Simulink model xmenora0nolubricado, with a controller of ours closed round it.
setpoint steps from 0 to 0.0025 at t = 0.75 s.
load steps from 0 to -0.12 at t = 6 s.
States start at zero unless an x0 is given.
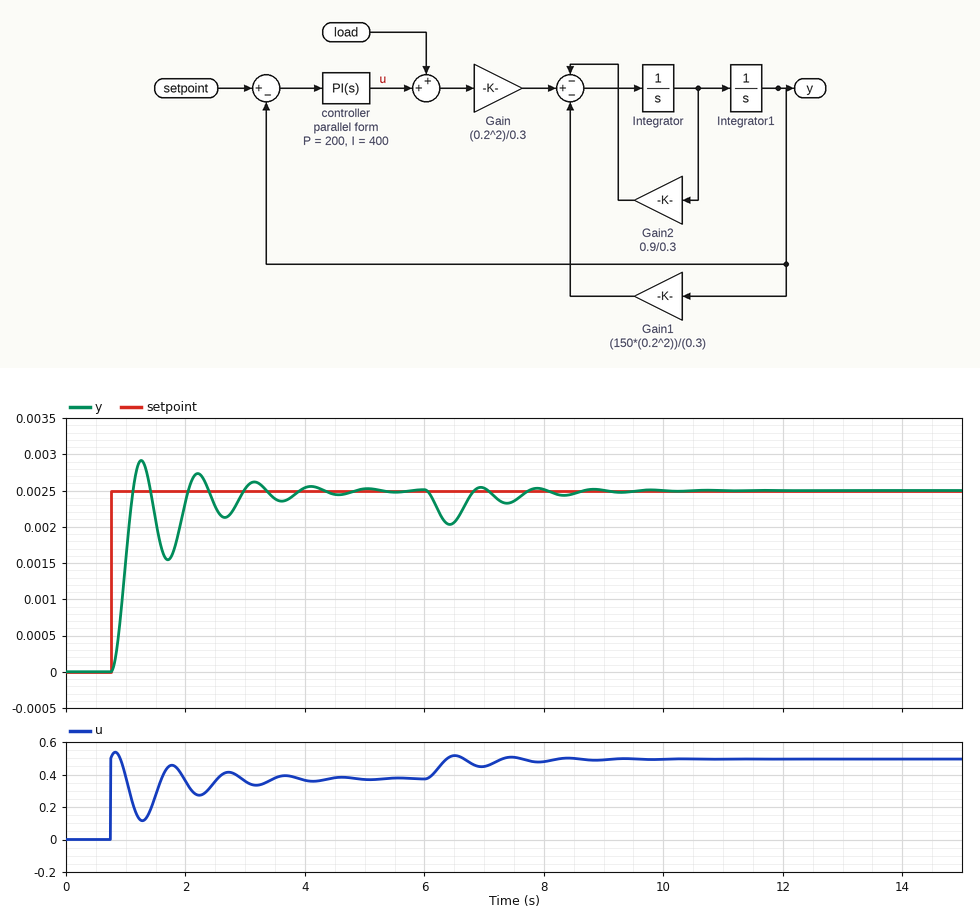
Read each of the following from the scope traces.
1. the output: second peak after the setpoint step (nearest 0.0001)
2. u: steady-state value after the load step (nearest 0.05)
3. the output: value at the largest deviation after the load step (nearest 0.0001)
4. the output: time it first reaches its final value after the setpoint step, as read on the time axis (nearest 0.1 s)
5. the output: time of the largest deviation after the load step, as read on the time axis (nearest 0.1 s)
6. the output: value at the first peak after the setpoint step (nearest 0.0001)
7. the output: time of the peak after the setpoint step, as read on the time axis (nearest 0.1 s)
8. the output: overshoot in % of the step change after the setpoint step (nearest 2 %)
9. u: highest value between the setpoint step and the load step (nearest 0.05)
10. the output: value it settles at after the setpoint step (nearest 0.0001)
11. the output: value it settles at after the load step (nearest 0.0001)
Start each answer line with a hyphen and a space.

- 0.0027
- 0.50
- 0.0020
- 1.1 s
- 6.4 s
- 0.0029
- 1.3 s
- 16 %
- 0.55
- 0.0025
- 0.0025
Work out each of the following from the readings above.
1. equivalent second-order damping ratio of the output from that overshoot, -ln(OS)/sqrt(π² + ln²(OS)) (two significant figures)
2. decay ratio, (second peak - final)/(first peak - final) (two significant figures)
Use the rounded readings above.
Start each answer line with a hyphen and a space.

- 0.50
- 0.50
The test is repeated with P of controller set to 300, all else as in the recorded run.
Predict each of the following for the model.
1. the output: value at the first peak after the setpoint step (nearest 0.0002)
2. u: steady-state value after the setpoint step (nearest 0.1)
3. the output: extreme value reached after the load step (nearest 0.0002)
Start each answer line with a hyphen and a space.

- 0.0030
- 0.4
- 0.0022
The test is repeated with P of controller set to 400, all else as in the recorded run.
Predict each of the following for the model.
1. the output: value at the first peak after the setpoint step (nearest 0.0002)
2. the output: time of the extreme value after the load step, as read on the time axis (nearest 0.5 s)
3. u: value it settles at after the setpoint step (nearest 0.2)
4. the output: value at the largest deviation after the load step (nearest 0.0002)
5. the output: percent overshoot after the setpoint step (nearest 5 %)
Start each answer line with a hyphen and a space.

- 0.0032
- 6.5 s
- 0.4
- 0.0022
- 30 %
